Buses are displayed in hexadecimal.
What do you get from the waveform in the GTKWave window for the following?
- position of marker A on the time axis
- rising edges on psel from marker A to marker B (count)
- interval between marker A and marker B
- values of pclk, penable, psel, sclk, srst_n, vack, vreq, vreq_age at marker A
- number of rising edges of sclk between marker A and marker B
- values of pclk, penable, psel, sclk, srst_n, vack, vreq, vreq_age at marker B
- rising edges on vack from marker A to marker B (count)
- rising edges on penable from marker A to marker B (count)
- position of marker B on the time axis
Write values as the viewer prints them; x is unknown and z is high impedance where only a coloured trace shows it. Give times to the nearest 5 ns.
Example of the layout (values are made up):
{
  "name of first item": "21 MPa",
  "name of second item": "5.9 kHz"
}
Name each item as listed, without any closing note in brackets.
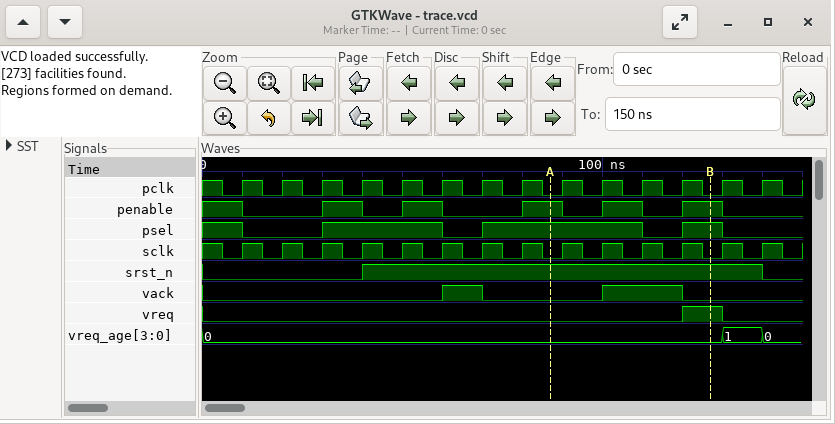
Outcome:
{
  "position of marker A on the time axis": "85 ns",
  "rising edges on psel from marker A to marker B": "1",
  "interval between marker A and marker B": "40 ns",
  "values of pclk, penable, psel, sclk, srst_n, vack, vreq, vreq_age at marker A": "pclk=0, penable=1, psel=1, sclk=0, srst_n=1, vack=0, vreq=0, vreq_age=0",
  "number of rising edges of sclk between marker A and marker B": "4",
  "values of pclk, penable, psel, sclk, srst_n, vack, vreq, vreq_age at marker B": "pclk=0, penable=1, psel=1, sclk=0, srst_n=1, vack=0, vreq=1, vreq_age=0",
  "rising edges on vack from marker A to marker B": "1",
  "rising edges on penable from marker A to marker B": "2",
  "position of marker B on the time axis": "125 ns"
}
